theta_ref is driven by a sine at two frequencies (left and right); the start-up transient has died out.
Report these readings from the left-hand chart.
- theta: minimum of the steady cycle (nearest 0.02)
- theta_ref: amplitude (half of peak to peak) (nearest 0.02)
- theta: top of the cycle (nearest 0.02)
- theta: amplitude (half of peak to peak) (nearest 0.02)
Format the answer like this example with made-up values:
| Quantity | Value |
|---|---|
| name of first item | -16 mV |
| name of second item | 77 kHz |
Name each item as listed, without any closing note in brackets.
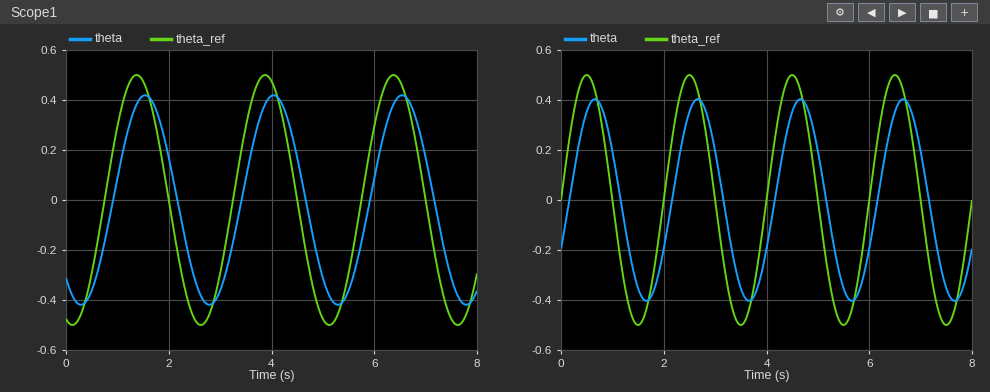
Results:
| Quantity | Value |
|---|---|
| theta: minimum of the steady cycle | -0.42 |
| theta_ref: amplitude (half of peak to peak) | 0.50 |
| theta: top of the cycle | 0.42 |
| theta: amplitude (half of peak to peak) | 0.42 |
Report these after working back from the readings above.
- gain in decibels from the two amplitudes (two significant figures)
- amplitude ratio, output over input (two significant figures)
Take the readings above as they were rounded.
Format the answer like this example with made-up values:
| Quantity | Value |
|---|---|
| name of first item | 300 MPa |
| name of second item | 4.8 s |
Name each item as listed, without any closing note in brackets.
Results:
| Quantity | Value |
|---|---|
| gain in decibels from the two amplitudes | -1.5 dB |
| amplitude ratio, output over input | 0.84 |
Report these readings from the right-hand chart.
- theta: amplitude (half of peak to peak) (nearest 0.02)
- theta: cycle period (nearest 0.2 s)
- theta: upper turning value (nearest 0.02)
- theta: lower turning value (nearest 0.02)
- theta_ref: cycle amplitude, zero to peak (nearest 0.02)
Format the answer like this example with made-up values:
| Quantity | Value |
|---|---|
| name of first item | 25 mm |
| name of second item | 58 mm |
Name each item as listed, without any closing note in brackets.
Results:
| Quantity | Value |
|---|---|
| theta: amplitude (half of peak to peak) | 0.40 |
| theta: cycle period | 2.0 s |
| theta: upper turning value | 0.40 |
| theta: lower turning value | -0.40 |
| theta_ref: cycle amplitude, zero to peak | 0.50 |
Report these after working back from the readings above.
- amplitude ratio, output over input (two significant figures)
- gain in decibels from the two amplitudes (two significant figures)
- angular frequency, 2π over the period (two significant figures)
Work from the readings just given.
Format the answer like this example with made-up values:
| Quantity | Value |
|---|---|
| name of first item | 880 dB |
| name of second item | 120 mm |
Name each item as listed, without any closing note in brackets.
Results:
| Quantity | Value |
|---|---|
| amplitude ratio, output over input | 0.80 |
| gain in decibels from the two amplitudes | -1.9 dB |
| angular frequency, 2π over the period | 3.1 rad/s |
